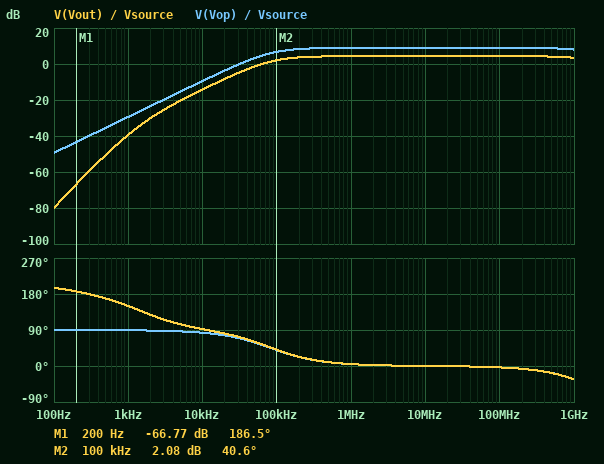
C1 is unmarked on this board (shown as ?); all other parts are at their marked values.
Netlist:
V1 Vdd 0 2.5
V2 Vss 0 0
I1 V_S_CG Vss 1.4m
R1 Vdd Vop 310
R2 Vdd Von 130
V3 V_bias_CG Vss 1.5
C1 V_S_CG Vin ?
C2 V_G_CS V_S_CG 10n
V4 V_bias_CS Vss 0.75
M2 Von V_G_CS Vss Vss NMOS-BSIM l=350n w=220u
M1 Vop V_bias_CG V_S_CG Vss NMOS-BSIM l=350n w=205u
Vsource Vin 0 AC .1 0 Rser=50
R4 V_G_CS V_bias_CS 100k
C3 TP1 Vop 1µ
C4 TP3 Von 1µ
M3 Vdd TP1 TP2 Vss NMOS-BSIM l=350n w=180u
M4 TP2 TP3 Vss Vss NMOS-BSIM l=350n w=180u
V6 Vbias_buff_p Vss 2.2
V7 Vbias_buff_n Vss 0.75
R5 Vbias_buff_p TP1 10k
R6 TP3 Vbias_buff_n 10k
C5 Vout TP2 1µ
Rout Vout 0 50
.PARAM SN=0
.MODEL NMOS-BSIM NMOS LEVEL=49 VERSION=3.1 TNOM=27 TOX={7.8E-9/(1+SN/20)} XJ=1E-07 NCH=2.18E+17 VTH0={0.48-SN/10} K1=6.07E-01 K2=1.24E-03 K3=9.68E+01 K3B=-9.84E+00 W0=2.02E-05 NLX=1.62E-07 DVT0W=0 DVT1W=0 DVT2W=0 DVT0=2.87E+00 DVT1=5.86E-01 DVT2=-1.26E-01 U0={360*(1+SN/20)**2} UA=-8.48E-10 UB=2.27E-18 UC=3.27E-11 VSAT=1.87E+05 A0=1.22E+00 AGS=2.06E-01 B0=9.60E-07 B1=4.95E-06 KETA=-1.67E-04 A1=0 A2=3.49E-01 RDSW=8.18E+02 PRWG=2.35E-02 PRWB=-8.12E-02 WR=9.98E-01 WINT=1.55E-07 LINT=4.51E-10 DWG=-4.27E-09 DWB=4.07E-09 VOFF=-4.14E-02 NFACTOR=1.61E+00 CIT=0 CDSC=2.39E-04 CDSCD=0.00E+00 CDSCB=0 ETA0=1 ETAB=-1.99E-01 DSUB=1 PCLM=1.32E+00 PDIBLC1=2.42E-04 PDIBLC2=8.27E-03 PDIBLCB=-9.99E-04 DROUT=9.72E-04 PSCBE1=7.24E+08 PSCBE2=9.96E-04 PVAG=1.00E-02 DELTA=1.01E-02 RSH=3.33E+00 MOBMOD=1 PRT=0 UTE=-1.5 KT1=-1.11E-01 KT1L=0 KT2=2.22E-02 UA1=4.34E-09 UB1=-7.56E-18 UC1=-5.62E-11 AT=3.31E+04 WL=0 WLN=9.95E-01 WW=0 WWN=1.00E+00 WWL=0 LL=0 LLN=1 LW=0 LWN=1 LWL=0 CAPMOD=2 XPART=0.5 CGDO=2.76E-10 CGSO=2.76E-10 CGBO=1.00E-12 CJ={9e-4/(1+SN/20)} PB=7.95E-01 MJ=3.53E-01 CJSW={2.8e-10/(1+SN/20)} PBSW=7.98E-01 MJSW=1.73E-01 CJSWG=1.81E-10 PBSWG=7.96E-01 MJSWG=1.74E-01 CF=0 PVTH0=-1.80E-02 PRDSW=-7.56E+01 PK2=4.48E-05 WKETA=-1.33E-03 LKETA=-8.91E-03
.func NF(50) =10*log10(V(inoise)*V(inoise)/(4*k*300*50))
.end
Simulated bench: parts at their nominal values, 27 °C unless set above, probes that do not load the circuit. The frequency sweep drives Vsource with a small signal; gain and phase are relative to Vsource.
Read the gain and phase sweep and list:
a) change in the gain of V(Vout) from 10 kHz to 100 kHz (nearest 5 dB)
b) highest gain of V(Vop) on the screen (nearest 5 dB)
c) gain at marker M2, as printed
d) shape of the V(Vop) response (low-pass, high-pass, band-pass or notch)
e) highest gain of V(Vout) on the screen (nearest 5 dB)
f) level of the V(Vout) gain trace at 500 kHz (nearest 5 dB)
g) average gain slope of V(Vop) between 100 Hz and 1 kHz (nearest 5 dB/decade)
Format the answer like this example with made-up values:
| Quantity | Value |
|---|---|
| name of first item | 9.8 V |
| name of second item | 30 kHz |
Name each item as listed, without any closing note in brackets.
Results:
| Quantity | Value |
|---|---|
| change in the gain of V(Vout) from 10 kHz to 100 kHz | 15 dB |
| highest gain of V(Vop) on the screen | 10 dB |
| gain at marker M2, as printed | 2.08 dB |
| shape of the V(Vop) response | high-pass |
| highest gain of V(Vout) on the screen | 5 dB |
| level of the V(Vout) gain trace at 500 kHz | 5 dB |
| average gain slope of V(Vop) between 100 Hz and 1 kHz | 20 dB/decade |
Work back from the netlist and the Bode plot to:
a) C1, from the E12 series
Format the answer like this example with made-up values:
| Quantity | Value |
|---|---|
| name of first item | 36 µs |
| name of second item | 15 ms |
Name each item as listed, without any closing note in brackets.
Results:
| Quantity | Value |
|---|---|
| C1, from the E12 series | 18 nF |
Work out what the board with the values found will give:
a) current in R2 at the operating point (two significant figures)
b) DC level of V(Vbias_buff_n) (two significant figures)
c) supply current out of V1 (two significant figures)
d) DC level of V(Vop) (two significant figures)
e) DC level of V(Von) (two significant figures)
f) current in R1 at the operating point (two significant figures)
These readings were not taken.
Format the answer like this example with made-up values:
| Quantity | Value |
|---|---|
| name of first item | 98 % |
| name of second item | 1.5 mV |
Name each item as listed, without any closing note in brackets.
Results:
| Quantity | Value |
|---|---|
| current in R2 at the operating point | 2.1 mA |
| DC level of V(Vbias_buff_n) | 750 mV |
| supply current out of V1 | 4.9 mA |
| DC level of V(Vop) | 2.1 V |
| DC level of V(Von) | 2.2 V |
| current in R1 at the operating point | 1.4 mA |
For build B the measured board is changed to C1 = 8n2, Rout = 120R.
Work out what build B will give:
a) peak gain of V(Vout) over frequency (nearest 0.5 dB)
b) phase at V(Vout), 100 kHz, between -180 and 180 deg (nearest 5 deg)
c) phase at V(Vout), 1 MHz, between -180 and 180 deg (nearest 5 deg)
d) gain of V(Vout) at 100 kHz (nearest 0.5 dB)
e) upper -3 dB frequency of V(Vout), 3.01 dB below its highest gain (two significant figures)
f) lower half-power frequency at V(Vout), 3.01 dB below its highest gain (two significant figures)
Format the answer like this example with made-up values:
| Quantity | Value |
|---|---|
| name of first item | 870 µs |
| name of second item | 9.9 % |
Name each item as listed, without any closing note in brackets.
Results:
| Quantity | Value |
|---|---|
| peak gain of V(Vout) over frequency | 7.5 dB |
| phase at V(Vout), 100 kHz, between -180 and 180 deg | 60 deg |
| phase at V(Vout), 1 MHz, between -180 and 180 deg | 10 deg |
| gain of V(Vout) at 100 kHz | 1.0 dB |
| upper -3 dB frequency of V(Vout), 3.01 dB below its highest gain | 2.4 GHz |
| lower half-power frequency at V(Vout), 3.01 dB below its highest gain | 180 kHz |
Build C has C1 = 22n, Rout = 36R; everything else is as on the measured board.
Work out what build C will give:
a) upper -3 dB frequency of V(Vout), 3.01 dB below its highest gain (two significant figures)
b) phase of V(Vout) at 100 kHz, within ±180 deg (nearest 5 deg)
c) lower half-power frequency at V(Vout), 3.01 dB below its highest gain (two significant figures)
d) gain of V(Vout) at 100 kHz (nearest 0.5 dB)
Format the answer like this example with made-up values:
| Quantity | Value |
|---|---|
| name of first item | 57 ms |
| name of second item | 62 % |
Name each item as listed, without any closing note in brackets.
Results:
| Quantity | Value |
|---|---|
| upper -3 dB frequency of V(Vout), 3.01 dB below its highest gain | 2.0 GHz |
| phase of V(Vout) at 100 kHz, within ±180 deg | 35 deg |
| lower half-power frequency at V(Vout), 3.01 dB below its highest gain | 68 kHz |
| gain of V(Vout) at 100 kHz | 1.0 dB |
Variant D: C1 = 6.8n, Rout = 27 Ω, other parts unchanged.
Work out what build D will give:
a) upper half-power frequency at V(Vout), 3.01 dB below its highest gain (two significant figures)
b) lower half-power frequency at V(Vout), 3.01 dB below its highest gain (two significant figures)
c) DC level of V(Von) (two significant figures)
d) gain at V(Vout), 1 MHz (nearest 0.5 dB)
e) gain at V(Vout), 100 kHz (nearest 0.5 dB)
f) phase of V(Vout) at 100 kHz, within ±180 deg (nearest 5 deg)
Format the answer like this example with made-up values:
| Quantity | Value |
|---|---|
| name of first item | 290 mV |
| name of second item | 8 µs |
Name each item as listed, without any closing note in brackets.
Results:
| Quantity | Value |
|---|---|
| upper half-power frequency at V(Vout), 3.01 dB below its highest gain | 1.9 GHz |
| lower half-power frequency at V(Vout), 3.01 dB below its highest gain | 220 kHz |
| DC level of V(Von) | 2.2 V |
| gain at V(Vout), 1 MHz | 1.0 dB |
| gain at V(Vout), 100 kHz | -6.5 dB |
| phase of V(Vout) at 100 kHz, within ±180 deg | 65 deg |
